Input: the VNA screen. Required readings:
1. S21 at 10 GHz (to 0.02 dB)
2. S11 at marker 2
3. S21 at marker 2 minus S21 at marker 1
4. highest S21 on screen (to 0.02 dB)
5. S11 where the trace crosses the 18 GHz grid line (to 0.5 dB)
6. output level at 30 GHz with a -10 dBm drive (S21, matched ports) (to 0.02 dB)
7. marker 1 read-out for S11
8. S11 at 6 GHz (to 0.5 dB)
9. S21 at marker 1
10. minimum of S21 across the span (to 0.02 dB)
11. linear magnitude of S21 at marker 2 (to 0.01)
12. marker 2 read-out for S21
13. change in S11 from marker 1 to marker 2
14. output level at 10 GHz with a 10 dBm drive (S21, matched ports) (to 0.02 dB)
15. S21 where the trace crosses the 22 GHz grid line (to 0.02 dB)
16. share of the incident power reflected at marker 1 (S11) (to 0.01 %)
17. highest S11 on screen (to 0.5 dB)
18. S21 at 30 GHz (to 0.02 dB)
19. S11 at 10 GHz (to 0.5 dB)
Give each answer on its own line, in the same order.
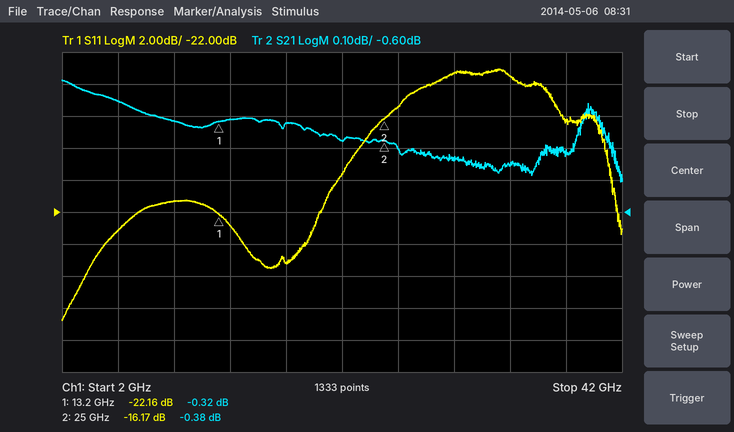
-0.32 dB
-16.17 dB
-0.06 dB
-0.18 dB
-25.0 dB
-10.44 dBm
-22.16 dB
-23.0 dB
-0.32 dB
-0.50 dB
0.96
-0.38 dB
5.99 dB
9.68 dBm
-0.38 dB
0.61 %
-13.0 dB
-0.44 dB
-21.5 dB
